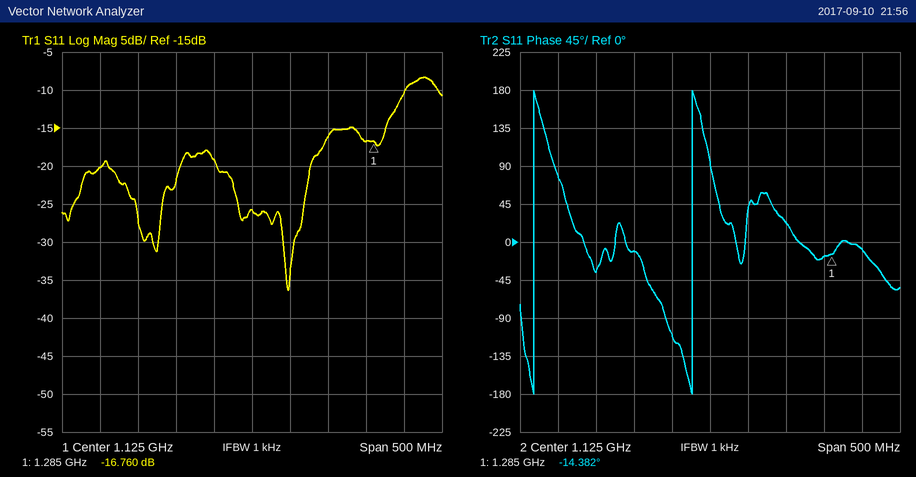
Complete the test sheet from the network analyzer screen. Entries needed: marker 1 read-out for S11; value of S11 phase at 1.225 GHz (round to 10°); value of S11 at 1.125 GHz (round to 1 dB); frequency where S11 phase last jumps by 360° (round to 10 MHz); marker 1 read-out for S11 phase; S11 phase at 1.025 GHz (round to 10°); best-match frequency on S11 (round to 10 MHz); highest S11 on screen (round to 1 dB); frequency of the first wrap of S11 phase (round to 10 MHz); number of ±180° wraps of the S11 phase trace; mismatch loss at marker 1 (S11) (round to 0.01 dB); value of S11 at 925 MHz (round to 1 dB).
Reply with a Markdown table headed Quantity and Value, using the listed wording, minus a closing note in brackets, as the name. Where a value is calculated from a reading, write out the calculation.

| Quantity | Value |
|---|---|
| marker 1 read-out for S11 | -16.760 dB |
| value of S11 phase at 1.225 GHz | 20° |
| value of S11 at 1.125 GHz | -26 dB |
| frequency where S11 phase last jumps by 360° | 1.10 GHz |
| marker 1 read-out for S11 phase | -14.382° |
| S11 phase at 1.025 GHz | -10° |
| best-match frequency on S11 | 1.17 GHz |
| highest S11 on screen | -8 dB |
| frequency of the first wrap of S11 phase | 890 MHz |
| number of ±180° wraps of the S11 phase trace | 2 |
| mismatch loss at marker 1 (S11) | −10 log10(1 − 10^(-16.76/10)) ≈ 0.09 dB |
| value of S11 at 925 MHz | -20 dB |
